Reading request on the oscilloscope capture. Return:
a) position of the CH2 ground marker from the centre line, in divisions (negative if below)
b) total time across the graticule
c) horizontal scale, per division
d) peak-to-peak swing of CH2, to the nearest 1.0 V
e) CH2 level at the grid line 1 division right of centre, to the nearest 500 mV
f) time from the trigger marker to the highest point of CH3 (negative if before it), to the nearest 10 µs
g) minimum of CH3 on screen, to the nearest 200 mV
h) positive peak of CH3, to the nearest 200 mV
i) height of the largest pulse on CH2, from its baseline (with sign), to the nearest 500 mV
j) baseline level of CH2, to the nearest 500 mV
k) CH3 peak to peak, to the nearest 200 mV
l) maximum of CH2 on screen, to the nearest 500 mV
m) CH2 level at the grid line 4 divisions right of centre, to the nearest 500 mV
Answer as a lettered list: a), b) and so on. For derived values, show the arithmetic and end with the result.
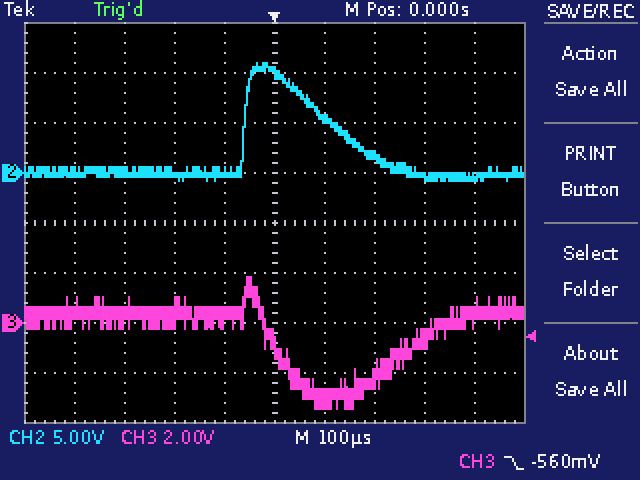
a) +1.0 div
b) 1 ms
c) 100 µs
d) 12.0 V
e) 5.5 V
f) -50 µs
g) -3.4 V
h) 1.8 V
i) 11.0 V − (0.0 V) = +11.0 V
j) 0.0 V
k) 1.8 V − (-3.4 V) = 5.2 V
l) 11.0 V
m) -500 mV
